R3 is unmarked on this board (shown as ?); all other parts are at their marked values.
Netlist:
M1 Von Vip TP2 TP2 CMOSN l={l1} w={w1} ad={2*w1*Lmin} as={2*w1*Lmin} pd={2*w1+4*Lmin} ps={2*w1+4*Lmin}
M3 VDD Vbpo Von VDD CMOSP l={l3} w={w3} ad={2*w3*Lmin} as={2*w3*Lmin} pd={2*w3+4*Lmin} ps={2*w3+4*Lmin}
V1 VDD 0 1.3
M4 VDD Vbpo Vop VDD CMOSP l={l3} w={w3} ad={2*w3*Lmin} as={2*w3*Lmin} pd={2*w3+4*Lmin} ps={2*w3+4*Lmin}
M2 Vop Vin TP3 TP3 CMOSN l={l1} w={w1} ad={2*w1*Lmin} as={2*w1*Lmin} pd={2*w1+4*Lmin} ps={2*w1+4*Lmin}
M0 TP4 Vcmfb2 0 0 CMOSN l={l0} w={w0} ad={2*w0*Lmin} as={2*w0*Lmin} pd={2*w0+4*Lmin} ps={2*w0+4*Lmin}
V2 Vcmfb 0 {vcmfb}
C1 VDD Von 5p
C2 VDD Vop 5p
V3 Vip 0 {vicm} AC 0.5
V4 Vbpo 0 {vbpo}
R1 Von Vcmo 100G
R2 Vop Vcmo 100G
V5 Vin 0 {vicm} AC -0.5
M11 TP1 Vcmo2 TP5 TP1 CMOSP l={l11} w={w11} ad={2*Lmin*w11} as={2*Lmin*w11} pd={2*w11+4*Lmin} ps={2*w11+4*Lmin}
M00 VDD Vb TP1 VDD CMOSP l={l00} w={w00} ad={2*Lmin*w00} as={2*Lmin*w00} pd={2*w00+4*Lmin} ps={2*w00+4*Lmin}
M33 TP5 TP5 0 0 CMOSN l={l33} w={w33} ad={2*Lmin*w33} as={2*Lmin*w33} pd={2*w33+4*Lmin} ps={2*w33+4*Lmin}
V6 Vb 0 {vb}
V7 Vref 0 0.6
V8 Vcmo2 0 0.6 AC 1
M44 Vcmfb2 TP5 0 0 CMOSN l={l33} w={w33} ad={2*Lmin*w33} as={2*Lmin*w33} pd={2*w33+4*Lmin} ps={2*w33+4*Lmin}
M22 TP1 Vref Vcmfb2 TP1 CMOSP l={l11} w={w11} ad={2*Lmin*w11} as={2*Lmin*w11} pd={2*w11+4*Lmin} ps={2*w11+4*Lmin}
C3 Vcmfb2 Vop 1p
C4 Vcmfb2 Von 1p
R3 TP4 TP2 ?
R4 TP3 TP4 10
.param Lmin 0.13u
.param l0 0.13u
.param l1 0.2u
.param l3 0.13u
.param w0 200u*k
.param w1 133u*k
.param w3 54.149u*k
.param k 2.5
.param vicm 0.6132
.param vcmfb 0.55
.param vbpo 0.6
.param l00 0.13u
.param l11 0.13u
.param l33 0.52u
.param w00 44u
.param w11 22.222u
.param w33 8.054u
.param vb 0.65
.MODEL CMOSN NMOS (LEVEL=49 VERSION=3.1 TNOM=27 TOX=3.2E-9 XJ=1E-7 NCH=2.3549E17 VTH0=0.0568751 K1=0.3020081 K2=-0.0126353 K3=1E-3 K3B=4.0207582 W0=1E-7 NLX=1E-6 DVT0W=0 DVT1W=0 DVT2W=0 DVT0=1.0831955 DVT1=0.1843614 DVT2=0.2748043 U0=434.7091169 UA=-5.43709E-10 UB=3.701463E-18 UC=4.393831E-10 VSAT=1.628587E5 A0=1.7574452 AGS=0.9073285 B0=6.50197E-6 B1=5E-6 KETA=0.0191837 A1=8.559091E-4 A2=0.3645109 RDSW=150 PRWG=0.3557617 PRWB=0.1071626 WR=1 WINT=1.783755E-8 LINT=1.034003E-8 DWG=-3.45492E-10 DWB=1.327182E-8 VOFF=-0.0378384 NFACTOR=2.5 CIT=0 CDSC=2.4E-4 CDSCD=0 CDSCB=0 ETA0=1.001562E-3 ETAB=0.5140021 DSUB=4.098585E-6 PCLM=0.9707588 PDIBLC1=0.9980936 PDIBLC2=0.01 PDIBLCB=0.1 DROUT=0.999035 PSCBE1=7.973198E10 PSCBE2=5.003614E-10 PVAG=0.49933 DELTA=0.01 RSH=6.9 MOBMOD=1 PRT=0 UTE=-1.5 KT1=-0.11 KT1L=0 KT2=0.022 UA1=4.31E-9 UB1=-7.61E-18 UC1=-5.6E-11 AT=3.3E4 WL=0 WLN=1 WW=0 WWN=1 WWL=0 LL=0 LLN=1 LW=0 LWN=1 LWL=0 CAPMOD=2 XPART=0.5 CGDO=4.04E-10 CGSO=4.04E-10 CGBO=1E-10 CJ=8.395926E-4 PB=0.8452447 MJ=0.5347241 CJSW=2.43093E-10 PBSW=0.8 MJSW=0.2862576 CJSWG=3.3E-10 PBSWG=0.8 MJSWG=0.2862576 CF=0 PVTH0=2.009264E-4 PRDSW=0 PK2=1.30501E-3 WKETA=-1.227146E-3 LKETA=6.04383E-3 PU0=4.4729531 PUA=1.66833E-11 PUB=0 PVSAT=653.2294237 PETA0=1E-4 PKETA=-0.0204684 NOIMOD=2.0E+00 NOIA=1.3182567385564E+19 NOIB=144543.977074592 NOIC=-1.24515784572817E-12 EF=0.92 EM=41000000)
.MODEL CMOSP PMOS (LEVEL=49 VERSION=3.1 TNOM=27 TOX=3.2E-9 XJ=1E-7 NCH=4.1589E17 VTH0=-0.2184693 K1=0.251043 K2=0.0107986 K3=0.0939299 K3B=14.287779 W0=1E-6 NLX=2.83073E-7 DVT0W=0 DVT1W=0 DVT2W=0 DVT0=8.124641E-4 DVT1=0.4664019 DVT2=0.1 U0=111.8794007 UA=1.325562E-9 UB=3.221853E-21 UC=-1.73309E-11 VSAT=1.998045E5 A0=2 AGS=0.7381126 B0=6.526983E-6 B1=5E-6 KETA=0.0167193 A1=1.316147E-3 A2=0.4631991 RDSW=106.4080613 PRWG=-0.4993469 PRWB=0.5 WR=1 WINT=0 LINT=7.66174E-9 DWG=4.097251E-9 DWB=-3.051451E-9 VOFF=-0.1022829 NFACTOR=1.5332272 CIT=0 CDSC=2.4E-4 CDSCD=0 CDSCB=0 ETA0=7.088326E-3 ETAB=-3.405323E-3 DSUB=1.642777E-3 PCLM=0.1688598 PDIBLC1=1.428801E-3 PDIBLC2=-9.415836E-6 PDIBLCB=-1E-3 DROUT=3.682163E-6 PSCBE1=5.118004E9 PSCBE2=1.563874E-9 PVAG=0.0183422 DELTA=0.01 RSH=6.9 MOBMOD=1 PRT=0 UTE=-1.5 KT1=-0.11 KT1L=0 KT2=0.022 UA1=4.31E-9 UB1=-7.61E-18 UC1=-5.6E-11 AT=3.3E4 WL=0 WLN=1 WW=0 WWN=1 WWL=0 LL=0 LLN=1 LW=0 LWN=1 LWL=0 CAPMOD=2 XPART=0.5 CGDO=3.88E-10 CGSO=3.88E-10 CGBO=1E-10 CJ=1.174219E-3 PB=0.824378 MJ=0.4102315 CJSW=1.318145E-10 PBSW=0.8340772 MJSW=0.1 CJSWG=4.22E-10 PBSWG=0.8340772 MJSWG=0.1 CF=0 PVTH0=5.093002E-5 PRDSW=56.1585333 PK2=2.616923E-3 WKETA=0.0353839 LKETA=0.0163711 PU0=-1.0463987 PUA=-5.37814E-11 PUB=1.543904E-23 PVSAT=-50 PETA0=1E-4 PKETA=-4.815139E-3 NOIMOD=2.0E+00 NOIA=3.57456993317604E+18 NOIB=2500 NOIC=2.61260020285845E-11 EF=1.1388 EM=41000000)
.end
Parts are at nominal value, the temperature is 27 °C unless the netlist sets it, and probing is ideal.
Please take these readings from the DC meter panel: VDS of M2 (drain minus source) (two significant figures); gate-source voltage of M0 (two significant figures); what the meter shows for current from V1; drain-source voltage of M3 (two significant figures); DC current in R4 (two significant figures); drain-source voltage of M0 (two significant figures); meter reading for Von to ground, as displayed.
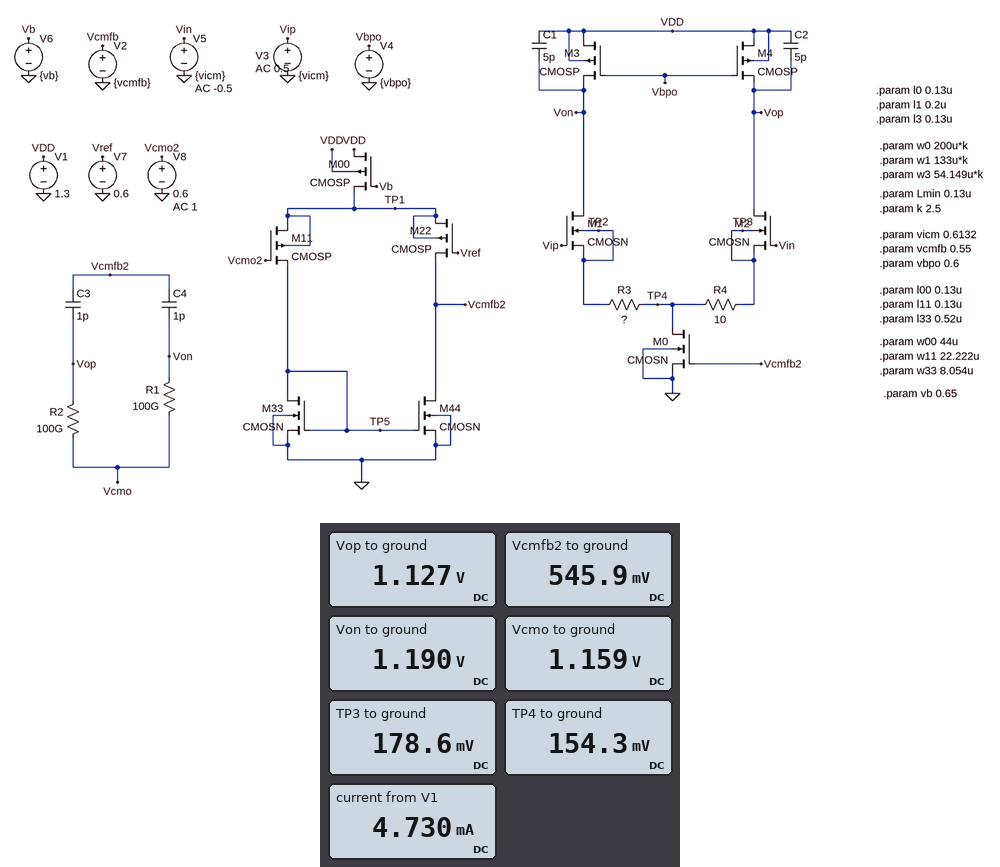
950 mV
550 mV
4.730 mA
110 mV
2.4 mA
150 mV
1.190 V
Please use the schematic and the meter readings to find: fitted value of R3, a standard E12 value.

27 Ω
